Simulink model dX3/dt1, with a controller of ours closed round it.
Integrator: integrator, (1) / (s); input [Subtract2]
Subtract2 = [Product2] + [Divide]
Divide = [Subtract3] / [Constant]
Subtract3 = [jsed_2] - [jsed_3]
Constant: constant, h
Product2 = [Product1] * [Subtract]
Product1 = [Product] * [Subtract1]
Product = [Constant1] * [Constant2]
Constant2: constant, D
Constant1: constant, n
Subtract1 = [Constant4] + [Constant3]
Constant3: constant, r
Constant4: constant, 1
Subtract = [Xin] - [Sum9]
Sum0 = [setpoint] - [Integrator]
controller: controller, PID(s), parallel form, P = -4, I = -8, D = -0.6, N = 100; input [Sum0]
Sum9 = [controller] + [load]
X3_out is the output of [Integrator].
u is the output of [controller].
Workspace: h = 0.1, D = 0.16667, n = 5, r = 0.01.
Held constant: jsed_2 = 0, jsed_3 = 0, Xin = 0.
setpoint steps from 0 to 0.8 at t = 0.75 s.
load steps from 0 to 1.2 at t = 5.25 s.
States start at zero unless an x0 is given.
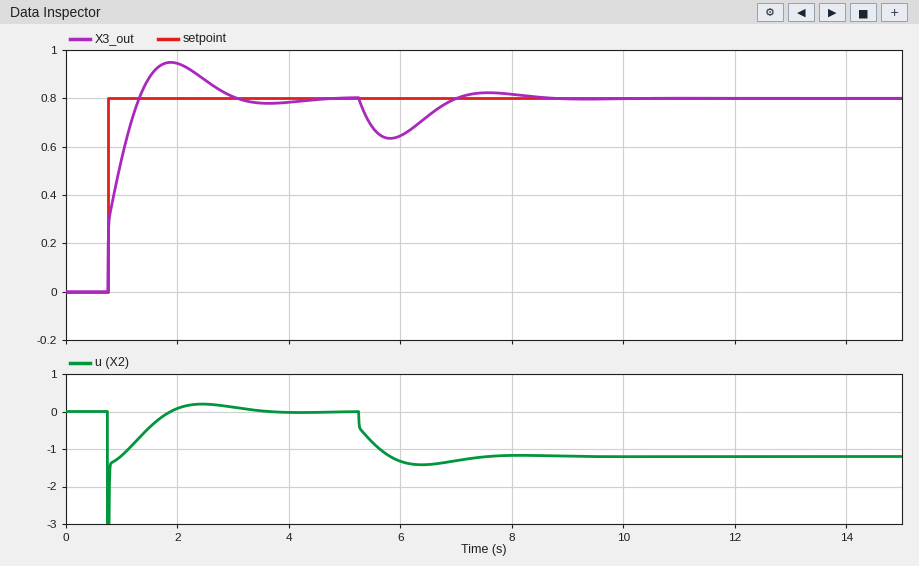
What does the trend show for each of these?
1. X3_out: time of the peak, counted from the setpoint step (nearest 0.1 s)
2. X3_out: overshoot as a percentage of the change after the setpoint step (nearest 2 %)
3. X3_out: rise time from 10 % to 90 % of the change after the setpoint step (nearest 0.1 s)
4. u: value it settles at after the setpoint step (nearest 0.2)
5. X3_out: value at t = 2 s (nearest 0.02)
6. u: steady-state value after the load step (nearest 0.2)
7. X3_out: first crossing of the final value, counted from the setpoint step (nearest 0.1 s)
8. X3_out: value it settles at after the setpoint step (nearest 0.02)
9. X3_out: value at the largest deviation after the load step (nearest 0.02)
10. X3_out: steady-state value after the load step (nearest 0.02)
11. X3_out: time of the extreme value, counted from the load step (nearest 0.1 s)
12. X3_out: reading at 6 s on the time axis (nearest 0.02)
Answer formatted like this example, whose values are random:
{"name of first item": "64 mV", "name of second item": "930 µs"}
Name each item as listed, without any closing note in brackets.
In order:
{"X3_out: time of the peak, counted from the setpoint step": "1.1 s", "X3_out: overshoot as a percentage of the change after the setpoint step": "18 %", "X3_out: rise time from 10 % to 90 % of the change after the setpoint step": "0.4 s", "u: value it settles at after the setpoint step": "0.0", "X3_out: value at t = 2 s": "0.94", "u: steady-state value after the load step": "-1.2", "X3_out: first crossing of the final value, counted from the setpoint step": "0.6 s", "X3_out: value it settles at after the setpoint step": "0.80", "X3_out: value at the largest deviation after the load step": "0.64", "X3_out: steady-state value after the load step": "0.80", "X3_out: time of the extreme value, counted from the load step": "0.6 s", "X3_out: reading at 6 s on the time axis": "0.64"}
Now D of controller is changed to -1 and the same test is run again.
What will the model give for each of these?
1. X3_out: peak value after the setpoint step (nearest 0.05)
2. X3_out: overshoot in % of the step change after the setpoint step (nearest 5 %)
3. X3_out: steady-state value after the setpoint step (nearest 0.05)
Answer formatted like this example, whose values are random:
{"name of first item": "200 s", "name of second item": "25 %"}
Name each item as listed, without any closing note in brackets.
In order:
{"X3_out: peak value after the setpoint step": "0.95", "X3_out: overshoot in % of the step change after the setpoint step": "15 %", "X3_out: steady-state value after the setpoint step": "0.80"}
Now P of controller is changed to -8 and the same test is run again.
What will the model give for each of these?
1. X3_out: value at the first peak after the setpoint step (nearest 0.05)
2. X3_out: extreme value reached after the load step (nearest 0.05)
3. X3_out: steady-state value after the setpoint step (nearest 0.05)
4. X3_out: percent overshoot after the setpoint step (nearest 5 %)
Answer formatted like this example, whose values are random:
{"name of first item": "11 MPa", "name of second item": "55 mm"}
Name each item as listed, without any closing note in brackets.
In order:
{"X3_out: value at the first peak after the setpoint step": "0.85", "X3_out: extreme value reached after the load step": "0.70", "X3_out: steady-state value after the setpoint step": "0.80", "X3_out: percent overshoot after the setpoint step": "10 %"}
